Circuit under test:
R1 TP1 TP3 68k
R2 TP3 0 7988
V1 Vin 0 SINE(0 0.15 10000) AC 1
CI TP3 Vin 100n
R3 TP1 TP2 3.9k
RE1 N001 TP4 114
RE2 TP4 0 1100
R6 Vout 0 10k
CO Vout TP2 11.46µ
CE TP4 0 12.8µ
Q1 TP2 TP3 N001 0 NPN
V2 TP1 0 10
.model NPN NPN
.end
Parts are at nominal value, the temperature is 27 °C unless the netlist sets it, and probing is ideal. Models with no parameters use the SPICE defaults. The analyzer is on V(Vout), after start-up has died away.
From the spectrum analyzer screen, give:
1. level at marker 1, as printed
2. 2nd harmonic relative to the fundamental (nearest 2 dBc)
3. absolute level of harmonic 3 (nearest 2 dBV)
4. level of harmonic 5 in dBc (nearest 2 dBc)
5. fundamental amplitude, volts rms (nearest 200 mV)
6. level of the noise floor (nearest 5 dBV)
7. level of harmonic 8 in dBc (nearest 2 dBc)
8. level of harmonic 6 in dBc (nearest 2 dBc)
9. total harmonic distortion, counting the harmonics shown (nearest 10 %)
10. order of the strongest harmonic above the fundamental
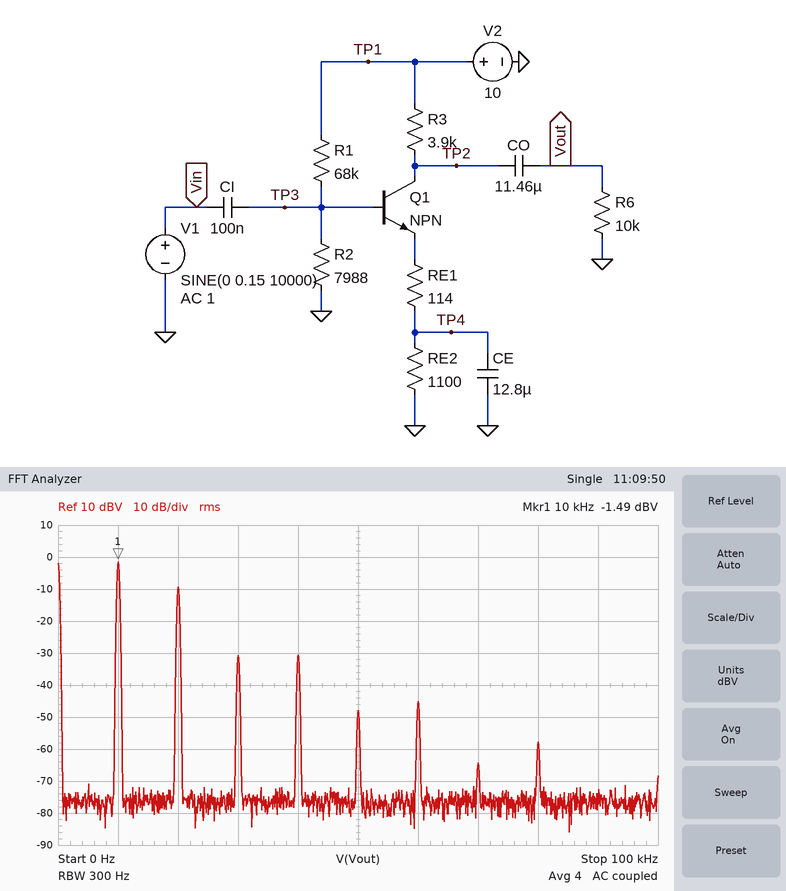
-1.49 dBV
-8 dBc
-30 dBV
-46 dBc
800 mV
-75 dBV
-56 dBc
-44 dBc
40 %
2
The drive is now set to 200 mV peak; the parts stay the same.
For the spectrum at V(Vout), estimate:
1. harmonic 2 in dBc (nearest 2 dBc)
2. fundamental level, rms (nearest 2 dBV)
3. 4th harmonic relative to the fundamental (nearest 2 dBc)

-6 dBc
0 dBV
-28 dBc
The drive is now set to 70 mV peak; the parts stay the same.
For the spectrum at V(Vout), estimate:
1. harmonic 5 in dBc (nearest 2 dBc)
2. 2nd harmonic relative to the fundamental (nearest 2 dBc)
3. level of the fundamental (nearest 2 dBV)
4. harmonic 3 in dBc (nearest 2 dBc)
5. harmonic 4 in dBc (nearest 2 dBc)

-58 dBc
-14 dBc
-6 dBV
-38 dBc
-48 dBc
